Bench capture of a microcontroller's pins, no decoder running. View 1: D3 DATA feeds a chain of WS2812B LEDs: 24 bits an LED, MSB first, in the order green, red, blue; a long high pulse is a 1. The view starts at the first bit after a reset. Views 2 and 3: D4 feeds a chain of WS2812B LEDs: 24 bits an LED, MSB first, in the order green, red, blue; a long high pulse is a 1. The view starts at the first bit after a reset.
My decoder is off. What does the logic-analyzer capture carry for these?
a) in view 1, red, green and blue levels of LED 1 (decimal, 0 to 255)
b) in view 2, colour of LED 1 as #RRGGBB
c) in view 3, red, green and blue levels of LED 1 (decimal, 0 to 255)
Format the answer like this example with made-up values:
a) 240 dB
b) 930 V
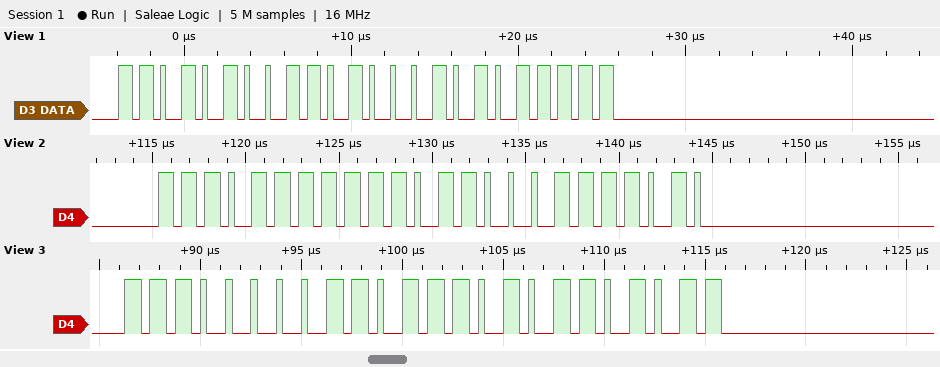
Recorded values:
a) 209, 212, 95
b) #ECEF7A
c) 221, 224, 107
